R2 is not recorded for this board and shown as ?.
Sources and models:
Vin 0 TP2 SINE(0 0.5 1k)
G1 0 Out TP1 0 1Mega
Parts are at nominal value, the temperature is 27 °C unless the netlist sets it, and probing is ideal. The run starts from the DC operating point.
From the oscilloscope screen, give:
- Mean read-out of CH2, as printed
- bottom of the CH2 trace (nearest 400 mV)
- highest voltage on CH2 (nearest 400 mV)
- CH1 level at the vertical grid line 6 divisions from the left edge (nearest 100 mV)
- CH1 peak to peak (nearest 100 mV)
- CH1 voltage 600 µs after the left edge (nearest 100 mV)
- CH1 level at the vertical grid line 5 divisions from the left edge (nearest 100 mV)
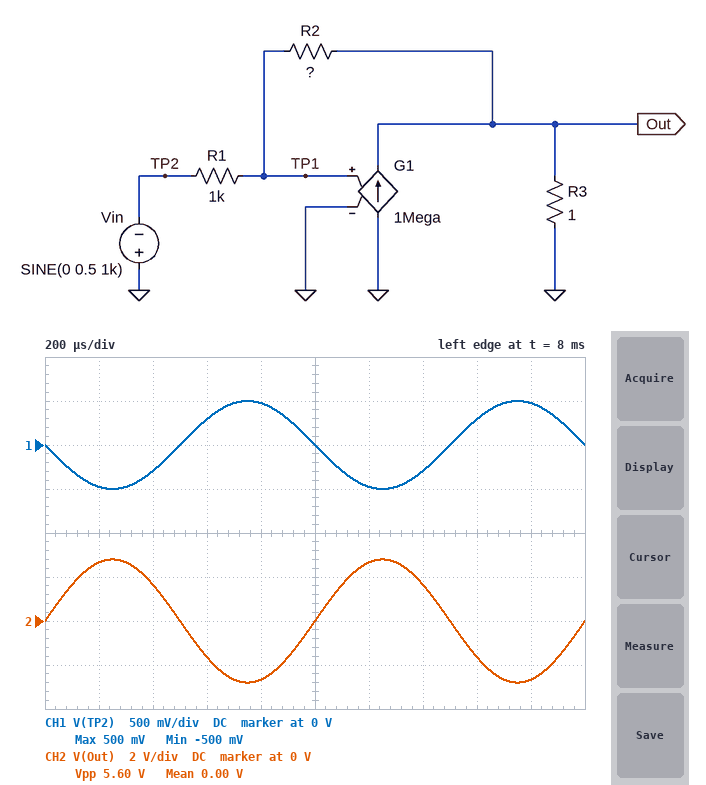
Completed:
0.00 V
-2.8 V
2.8 V
-500 mV
1.0 V
300 mV
0 V
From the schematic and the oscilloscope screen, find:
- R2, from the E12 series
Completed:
5.6 kΩ
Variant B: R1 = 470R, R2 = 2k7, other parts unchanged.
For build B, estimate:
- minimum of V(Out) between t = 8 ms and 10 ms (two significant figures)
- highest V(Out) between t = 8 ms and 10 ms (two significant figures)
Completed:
-2.9 V
2.9 V
